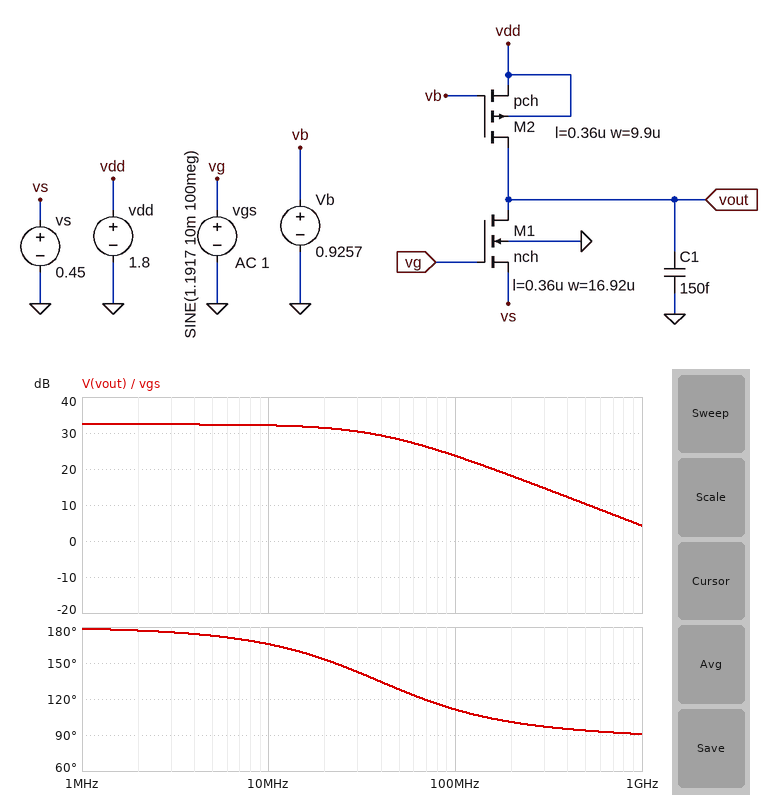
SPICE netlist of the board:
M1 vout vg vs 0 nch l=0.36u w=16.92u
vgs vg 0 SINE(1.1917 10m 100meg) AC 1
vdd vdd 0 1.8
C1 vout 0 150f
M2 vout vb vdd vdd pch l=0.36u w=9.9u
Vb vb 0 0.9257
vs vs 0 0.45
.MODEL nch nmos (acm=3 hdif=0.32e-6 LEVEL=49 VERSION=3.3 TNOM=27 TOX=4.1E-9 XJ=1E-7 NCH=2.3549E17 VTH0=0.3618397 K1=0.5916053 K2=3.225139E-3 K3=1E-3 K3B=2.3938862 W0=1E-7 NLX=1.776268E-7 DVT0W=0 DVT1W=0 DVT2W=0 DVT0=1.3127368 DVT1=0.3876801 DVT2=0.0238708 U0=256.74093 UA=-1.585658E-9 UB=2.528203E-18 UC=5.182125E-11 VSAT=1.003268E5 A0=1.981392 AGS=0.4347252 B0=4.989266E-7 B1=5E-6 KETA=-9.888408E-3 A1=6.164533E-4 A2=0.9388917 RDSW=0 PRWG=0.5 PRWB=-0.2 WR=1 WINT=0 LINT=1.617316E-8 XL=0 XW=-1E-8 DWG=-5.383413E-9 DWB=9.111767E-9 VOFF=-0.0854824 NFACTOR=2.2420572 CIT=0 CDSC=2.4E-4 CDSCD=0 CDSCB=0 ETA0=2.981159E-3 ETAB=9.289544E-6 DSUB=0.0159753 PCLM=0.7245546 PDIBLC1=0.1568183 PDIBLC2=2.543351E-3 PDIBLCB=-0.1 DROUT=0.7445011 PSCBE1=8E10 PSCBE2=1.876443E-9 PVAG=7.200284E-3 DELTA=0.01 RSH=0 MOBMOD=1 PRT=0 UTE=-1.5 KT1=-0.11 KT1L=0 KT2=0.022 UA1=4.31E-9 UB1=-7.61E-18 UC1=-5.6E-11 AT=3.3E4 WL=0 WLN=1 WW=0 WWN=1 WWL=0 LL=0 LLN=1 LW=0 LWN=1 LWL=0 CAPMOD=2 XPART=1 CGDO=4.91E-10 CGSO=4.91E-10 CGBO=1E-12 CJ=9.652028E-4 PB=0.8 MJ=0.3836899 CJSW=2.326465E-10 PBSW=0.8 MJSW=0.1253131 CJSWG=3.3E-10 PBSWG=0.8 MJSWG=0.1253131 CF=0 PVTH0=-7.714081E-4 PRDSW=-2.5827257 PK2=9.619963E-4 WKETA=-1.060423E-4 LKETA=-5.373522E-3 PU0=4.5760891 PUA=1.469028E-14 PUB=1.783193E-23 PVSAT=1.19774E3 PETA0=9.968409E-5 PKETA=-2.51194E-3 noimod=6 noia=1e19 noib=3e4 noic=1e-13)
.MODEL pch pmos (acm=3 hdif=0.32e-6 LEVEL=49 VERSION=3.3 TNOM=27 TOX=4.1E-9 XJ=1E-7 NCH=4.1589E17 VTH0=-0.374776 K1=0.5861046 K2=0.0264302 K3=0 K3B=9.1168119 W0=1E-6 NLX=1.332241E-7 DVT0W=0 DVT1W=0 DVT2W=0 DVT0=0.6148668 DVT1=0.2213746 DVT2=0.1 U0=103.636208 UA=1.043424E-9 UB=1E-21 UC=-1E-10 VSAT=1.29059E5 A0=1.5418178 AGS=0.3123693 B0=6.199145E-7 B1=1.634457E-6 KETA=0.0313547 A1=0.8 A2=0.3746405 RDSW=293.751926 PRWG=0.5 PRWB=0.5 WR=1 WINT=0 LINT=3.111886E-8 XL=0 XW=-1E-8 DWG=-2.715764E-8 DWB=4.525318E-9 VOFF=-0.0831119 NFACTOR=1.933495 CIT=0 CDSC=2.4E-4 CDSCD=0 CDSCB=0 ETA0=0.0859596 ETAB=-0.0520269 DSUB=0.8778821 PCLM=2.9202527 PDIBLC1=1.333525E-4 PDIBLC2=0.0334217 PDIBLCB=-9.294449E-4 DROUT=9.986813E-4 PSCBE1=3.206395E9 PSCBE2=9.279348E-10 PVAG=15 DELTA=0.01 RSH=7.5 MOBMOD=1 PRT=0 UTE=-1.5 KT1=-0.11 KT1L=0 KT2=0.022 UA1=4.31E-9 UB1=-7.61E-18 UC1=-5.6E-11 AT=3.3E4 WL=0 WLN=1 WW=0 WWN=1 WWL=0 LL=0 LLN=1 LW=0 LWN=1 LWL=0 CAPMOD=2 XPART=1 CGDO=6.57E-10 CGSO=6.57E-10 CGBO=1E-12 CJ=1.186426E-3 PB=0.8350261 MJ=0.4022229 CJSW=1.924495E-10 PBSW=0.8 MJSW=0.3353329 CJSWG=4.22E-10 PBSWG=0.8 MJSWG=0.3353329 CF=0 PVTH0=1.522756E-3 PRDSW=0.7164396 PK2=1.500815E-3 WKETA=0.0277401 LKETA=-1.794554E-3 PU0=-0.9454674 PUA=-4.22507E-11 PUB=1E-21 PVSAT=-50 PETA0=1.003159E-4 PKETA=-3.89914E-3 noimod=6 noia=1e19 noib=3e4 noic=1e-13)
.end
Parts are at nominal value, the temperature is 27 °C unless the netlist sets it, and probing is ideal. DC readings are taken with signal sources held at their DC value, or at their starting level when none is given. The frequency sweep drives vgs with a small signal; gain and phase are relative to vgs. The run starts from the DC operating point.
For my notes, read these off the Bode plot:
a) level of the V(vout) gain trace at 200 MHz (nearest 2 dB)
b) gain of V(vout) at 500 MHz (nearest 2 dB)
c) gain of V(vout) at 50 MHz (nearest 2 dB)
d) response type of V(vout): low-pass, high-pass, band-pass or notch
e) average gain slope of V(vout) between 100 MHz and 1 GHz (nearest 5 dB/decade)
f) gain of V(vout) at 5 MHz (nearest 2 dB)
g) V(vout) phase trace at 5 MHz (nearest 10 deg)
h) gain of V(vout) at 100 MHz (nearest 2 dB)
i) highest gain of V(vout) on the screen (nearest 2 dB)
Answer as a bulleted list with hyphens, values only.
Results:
- 18 dB
- 10 dB
- 28 dB
- low-pass
- -20 dB/decade
- 32 dB
- 170 deg
- 24 dB
- 32 dB
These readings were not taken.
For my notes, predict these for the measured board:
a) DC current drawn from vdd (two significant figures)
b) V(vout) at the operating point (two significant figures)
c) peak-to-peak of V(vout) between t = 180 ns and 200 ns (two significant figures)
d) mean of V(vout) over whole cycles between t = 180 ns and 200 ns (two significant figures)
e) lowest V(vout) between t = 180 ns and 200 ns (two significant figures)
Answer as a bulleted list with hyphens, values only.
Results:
- 170 µA
- 1.1 V
- 300 mV
- 1.1 V
- 940 mV
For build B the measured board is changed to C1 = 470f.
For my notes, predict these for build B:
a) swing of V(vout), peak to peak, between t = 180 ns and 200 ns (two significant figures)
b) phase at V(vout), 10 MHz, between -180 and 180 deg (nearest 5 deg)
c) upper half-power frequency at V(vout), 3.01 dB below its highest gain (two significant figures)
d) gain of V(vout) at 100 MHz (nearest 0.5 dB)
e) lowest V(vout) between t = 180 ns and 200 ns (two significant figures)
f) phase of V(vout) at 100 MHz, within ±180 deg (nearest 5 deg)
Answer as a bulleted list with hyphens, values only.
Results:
- 120 mV
- 145 deg
- 15 MHz
- 15.5 dB
- 1.0 V
- 100 deg
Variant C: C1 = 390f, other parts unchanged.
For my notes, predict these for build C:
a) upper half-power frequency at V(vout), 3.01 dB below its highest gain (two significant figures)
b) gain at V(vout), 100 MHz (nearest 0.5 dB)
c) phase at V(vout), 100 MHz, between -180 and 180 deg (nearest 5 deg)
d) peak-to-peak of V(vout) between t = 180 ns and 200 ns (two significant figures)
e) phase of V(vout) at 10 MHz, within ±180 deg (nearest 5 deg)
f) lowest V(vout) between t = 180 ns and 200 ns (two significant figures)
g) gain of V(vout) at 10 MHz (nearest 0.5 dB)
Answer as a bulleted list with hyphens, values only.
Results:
- 17 MHz
- 17.0 dB
- 100 deg
- 140 mV
- 150 deg
- 1.0 V
- 31.0 dB
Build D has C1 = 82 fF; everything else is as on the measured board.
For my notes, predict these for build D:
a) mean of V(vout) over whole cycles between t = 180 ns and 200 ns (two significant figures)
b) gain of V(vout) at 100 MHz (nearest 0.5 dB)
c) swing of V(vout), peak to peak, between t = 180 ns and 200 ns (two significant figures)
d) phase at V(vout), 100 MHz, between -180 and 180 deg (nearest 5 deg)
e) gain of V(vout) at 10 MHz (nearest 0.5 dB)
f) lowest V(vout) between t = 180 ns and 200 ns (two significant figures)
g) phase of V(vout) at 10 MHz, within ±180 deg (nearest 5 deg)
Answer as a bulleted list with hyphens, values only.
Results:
- 1.1 V
- 26.5 dB
- 430 mV
- 120 deg
- 32.5 dB
- 880 mV
- 170 deg
